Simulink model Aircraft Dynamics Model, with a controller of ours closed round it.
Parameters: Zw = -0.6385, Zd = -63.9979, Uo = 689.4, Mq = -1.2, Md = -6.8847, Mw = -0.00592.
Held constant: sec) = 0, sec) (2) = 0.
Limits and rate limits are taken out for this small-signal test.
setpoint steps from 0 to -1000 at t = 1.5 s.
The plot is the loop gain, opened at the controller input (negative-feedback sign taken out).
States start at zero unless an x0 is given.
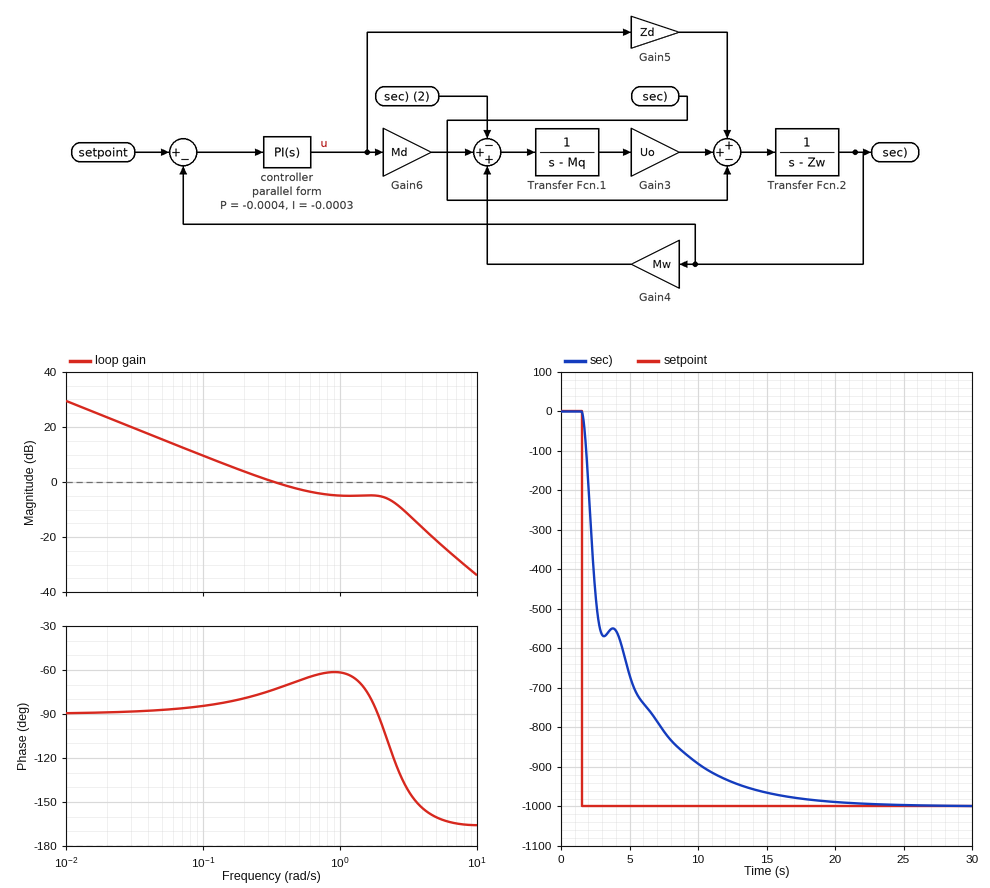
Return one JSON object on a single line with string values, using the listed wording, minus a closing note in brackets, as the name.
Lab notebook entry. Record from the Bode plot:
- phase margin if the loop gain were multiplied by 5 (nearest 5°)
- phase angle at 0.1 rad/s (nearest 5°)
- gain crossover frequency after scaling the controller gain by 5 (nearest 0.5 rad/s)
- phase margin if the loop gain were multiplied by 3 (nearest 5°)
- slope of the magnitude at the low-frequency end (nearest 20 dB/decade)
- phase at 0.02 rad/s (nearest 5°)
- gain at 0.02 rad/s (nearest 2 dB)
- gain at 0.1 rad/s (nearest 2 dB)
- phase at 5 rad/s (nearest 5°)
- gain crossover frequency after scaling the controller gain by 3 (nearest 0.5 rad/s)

{"phase margin if the loop gain were multiplied by 5": "30°", "phase angle at 0.1 rad/s": "-85°", "gain crossover frequency after scaling the controller gain by 5": "3.5 rad/s", "phase margin if the loop gain were multiplied by 3": "45°", "slope of the magnitude at the low-frequency end": "-20 dB/decade", "phase at 0.02 rad/s": "-90°", "gain at 0.02 rad/s": "24 dB", "gain at 0.1 rad/s": "10 dB", "phase at 5 rad/s": "-160°", "gain crossover frequency after scaling the controller gain by 3": "3.0 rad/s"}
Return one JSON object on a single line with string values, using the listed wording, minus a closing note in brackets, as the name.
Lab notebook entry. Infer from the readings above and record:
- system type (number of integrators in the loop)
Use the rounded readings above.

{"system type": "1"}
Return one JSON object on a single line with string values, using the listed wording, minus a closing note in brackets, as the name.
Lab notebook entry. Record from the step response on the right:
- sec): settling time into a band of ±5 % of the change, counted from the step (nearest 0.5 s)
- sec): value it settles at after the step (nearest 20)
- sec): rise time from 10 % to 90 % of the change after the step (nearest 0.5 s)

{"sec): settling time into a band of ±5 % of the change, counted from the step": "12.0 s", "sec): value it settles at after the step": "-1000", "sec): rise time from 10 % to 90 % of the change after the step": "8.5 s"}
